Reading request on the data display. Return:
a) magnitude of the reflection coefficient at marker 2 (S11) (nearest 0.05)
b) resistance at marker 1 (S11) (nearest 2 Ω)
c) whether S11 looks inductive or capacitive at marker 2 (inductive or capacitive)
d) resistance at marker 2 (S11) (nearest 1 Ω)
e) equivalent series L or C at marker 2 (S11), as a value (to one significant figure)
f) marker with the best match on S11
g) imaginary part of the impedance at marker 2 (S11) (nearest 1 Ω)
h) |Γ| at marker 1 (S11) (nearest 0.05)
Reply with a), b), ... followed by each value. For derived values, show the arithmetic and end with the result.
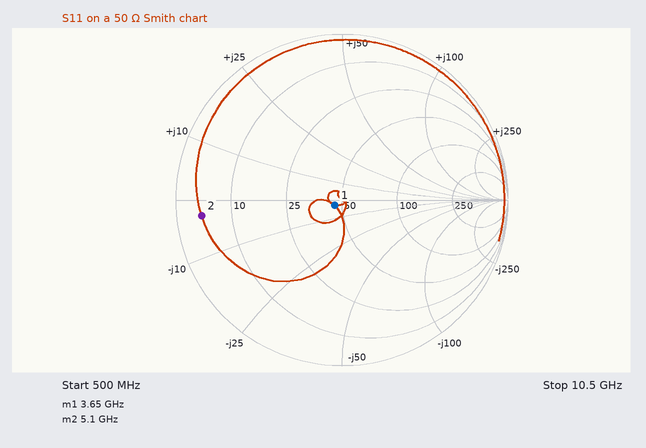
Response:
a) 0.85
b) 46 Ω
c) capacitive
d) 4 Ω
e) C = 1/(2π × 5.1 GHz × 3 Ω) ≈ 10 pF
f) marker 1
g) -3 Ω
h) 0.05
